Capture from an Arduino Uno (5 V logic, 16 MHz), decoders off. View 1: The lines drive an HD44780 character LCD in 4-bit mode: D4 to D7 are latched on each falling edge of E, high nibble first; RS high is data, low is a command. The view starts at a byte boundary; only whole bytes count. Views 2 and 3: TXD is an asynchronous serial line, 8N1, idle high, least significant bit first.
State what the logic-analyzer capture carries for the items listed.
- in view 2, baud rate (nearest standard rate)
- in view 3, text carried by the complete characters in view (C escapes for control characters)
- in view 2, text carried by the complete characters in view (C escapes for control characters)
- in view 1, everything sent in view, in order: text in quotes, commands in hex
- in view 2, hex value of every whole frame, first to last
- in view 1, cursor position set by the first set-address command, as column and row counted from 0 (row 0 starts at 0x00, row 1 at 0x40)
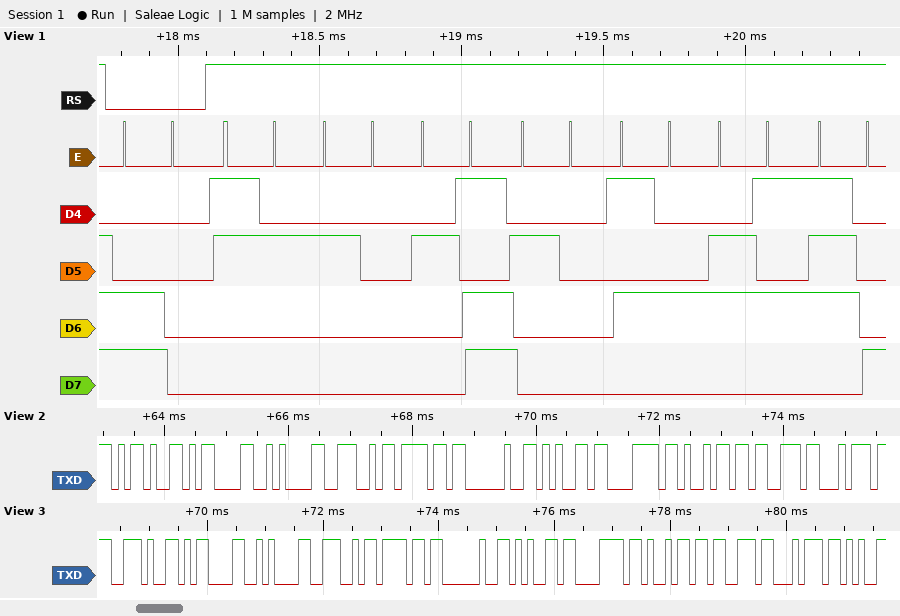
9600 baud
".\r\nNo exist"
"-\r\nNo exist"
0xC0 "2 - Tex"
2D 0D 0A 4E 6F 20 65 78 69 73 74
column 0, row 1
